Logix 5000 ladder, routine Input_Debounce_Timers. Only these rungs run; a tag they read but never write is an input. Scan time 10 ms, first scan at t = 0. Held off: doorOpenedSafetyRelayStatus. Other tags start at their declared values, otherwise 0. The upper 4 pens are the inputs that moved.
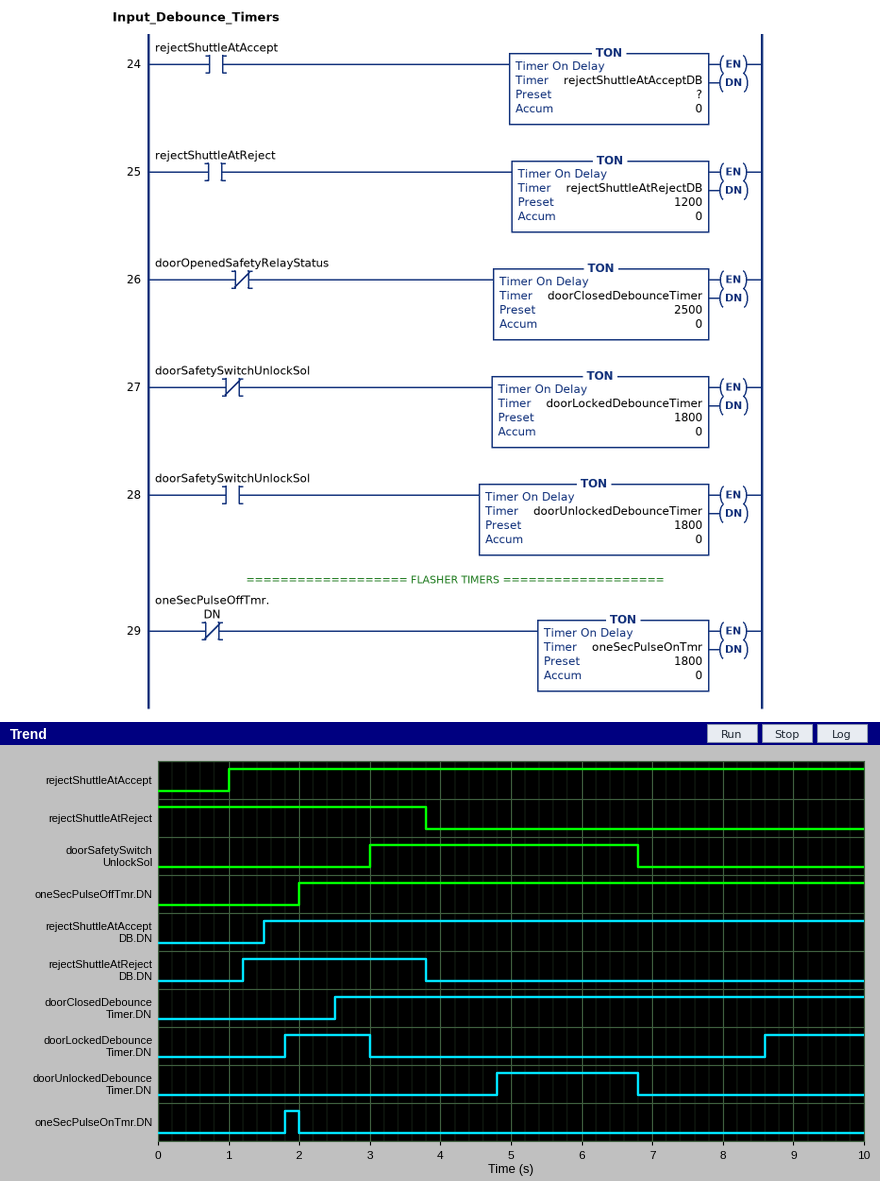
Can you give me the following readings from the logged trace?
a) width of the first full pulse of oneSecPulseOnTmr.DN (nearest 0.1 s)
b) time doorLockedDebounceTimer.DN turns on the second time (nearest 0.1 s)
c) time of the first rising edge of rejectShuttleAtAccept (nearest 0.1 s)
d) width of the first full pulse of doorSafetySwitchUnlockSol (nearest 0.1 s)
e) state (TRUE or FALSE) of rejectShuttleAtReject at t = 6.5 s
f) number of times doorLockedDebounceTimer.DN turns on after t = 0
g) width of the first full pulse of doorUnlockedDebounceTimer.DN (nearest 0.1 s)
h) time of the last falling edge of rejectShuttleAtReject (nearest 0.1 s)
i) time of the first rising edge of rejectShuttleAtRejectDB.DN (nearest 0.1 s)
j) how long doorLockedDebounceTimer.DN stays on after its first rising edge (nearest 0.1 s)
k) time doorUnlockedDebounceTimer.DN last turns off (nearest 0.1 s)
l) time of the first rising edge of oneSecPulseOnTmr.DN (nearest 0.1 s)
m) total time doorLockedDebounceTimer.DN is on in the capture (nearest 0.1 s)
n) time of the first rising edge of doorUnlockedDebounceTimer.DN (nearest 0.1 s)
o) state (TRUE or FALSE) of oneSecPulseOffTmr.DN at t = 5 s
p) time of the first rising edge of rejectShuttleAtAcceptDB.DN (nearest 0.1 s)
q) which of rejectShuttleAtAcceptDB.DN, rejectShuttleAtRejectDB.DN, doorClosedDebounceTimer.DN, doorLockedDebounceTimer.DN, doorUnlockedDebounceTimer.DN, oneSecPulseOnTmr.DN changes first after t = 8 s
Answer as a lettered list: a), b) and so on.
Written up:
a) 0.2 s
b) 8.6 s
c) 1.0 s
d) 3.8 s
e) FALSE
f) 2
g) 2.0 s
h) 3.8 s
i) 1.2 s
j) 1.2 s
k) 6.8 s
l) 1.8 s
m) 2.6 s
n) 4.8 s
o) TRUE
p) 1.5 s
q) doorLockedDebounceTimer.DN
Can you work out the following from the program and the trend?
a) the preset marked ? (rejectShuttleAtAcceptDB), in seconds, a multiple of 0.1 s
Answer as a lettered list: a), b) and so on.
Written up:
a) 0.5 s
